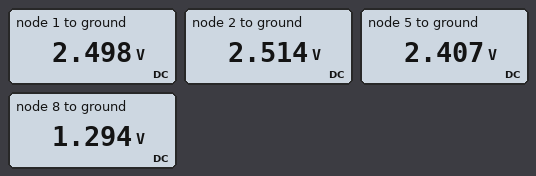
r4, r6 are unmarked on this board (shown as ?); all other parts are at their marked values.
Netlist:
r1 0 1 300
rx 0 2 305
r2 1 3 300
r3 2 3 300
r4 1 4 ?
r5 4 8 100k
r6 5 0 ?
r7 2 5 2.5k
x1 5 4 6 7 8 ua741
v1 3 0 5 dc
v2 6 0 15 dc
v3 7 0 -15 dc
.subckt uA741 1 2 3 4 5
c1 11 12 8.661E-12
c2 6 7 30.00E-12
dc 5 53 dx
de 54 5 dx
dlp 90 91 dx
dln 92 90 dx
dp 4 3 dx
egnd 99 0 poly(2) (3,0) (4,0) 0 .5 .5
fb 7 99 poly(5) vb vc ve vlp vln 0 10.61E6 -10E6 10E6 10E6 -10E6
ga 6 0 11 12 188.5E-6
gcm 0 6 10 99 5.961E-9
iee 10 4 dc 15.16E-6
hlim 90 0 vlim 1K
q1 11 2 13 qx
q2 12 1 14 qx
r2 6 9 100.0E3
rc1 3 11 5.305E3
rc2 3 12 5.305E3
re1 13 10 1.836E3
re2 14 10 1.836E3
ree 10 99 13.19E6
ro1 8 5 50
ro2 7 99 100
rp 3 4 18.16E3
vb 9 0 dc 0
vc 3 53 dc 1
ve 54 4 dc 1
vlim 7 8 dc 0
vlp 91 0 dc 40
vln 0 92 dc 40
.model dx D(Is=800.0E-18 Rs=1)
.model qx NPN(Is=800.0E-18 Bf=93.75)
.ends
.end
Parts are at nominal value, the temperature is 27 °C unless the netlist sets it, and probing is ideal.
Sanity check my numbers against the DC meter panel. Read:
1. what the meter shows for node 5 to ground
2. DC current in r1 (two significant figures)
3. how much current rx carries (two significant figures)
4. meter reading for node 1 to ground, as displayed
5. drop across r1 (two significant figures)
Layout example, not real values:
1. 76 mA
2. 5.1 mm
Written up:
1. 2.407 V
2. 8.3 mA
3. 8.2 mA
4. 2.498 V
5. 2.5 V
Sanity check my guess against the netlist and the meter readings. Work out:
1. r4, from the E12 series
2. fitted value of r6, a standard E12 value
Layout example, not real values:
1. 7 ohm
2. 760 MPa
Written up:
1. 8.2 kΩ
2. 56 kΩ
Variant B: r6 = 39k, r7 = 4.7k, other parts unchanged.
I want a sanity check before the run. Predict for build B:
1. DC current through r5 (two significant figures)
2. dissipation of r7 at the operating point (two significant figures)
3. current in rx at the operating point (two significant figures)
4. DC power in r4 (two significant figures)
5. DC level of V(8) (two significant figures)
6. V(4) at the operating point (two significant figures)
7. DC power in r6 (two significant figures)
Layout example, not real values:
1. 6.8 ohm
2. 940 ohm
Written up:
1. 31 µA
2. 16 µW
3. 8.2 mA
4. 7.9 µW
5. -850 mV
6. 2.2 V
7. 130 µW
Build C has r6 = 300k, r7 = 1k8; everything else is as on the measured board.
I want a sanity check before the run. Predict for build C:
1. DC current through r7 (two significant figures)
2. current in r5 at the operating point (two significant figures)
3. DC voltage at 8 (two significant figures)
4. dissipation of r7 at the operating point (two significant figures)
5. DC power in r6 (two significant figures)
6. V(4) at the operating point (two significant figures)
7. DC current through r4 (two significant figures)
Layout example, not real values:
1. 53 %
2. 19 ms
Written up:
1. 8.4 µA
2. 580 nA
3. 2.6 V
4. 130 nW
5. 21 µW
6. 2.5 V
7. 500 nA
